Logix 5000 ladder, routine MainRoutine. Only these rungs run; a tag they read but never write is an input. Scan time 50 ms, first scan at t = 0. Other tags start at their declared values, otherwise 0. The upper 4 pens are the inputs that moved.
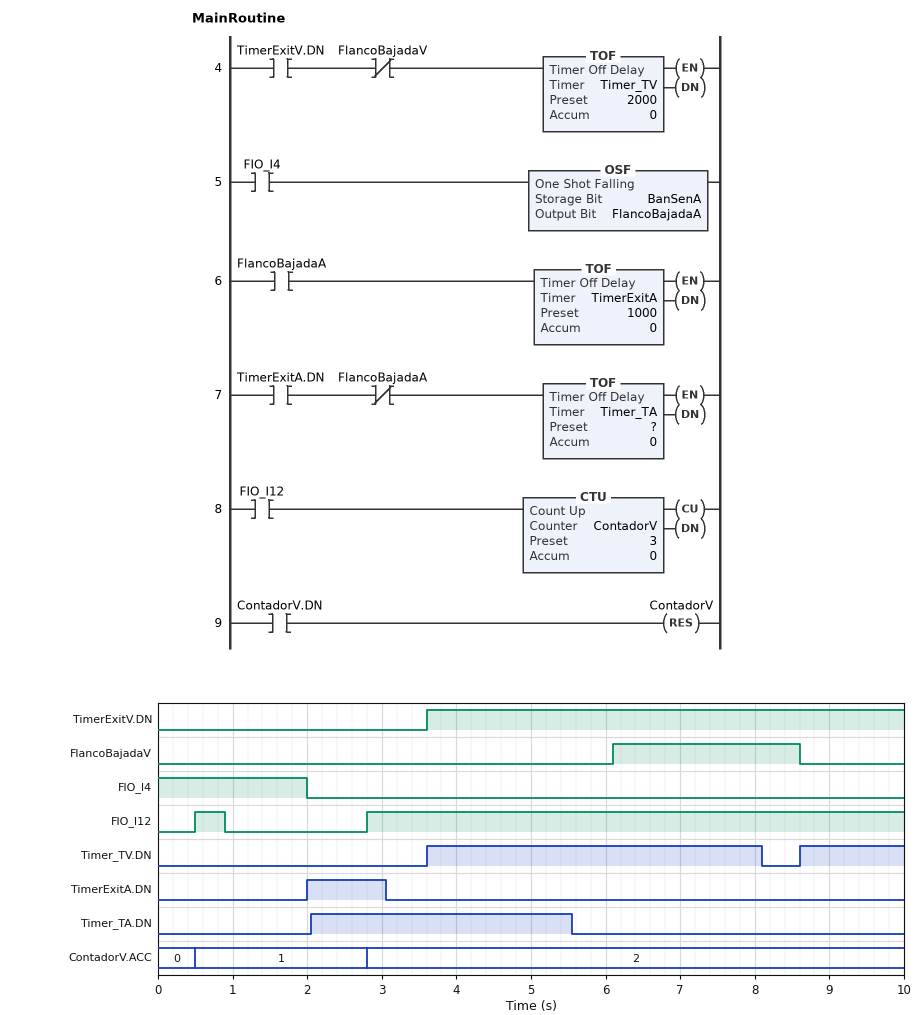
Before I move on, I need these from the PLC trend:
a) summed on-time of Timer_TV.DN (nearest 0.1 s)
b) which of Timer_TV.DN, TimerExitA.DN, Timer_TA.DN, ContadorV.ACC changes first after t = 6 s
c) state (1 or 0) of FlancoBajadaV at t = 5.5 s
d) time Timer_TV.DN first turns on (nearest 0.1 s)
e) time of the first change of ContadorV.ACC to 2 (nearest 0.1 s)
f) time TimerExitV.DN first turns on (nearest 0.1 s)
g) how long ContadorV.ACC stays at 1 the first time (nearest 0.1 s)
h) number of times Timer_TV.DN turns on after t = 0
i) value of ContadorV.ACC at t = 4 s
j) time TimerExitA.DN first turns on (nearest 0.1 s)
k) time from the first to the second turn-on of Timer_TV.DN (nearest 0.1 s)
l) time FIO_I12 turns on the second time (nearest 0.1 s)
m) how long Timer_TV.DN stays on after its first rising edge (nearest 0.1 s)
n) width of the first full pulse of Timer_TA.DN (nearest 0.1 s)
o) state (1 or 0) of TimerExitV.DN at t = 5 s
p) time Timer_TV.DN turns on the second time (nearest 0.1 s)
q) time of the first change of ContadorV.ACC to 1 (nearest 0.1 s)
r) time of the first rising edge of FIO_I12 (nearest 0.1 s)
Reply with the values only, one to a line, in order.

5.9 s
Timer_TV.DN
0
3.6 s
2.8 s
3.6 s
2.3 s
2
2
2.0 s
5.0 s
2.8 s
4.5 s
3.5 s
1
8.6 s
0.5 s
0.5 s
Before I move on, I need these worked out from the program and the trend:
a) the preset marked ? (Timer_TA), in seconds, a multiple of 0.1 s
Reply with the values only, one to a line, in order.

2.5 s
